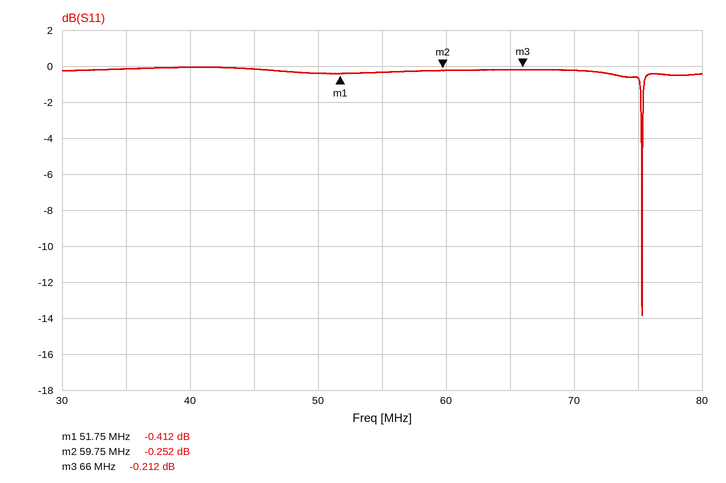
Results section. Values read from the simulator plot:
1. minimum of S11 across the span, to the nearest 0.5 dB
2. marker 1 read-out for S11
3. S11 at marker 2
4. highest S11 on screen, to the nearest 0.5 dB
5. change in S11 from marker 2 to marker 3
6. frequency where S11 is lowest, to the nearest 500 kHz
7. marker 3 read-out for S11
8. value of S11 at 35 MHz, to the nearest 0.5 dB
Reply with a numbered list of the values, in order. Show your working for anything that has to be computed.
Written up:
1. -14.0 dB
2. -0.412 dB
3. -0.252 dB
4. 0.0 dB
5. -0.212 − (-0.252) = 0.040 dB
6. 75.5 MHz
7. -0.212 dB
8. 0.0 dB
